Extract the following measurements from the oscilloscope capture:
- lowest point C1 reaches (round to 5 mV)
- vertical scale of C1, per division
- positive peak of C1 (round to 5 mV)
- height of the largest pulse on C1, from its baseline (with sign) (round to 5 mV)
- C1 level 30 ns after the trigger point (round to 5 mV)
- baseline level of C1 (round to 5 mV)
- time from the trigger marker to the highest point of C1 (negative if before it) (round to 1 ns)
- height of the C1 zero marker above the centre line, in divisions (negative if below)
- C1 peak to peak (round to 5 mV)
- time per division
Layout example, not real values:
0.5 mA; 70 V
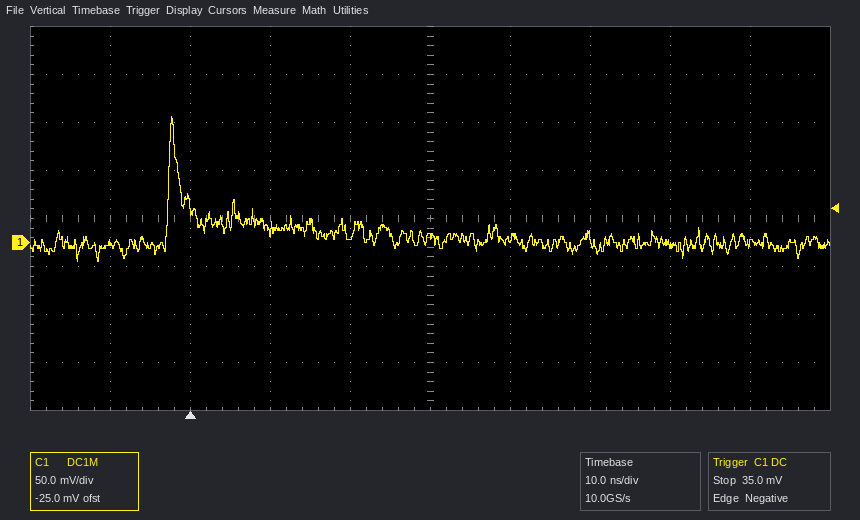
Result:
-20 mV; 50 mV; 130 mV; +130 mV; 5 mV; 0 mV; -2 ns; -0.5 div; 150 mV; 10 ns
